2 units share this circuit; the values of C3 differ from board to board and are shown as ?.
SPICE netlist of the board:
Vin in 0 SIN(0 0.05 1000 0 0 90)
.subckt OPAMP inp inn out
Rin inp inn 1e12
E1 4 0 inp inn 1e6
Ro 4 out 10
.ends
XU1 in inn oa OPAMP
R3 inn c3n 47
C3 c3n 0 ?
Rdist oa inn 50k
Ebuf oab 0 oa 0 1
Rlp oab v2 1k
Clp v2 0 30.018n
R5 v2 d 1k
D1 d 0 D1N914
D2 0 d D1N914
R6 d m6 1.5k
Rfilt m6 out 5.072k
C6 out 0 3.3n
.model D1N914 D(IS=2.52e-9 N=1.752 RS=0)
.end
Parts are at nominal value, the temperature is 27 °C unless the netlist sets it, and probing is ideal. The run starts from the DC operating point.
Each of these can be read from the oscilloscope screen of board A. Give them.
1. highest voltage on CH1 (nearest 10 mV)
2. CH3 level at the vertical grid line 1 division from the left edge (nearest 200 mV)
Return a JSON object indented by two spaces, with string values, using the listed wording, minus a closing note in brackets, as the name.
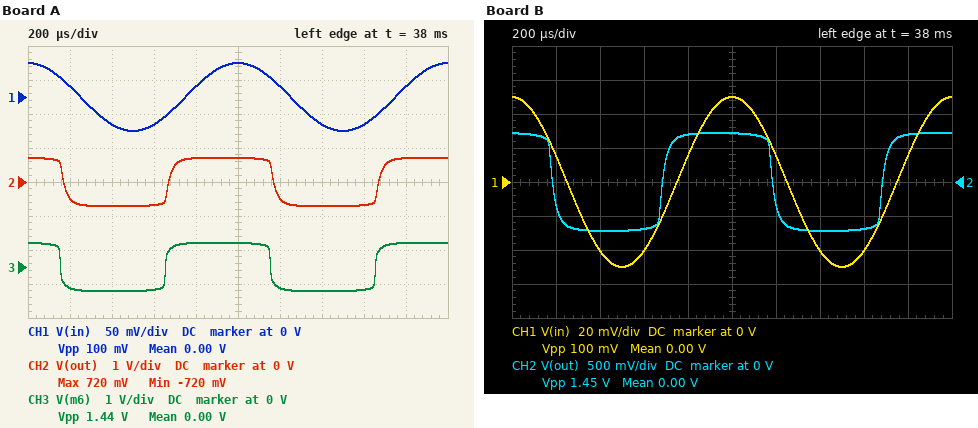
{
  "highest voltage on CH1": "50 mV",
  "CH3 level at the vertical grid line 1 division from the left edge": "-600 mV"
}
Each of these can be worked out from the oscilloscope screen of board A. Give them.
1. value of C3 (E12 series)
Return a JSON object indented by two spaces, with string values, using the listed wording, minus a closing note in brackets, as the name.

{
  "value of C3": "3.9 µF"
}
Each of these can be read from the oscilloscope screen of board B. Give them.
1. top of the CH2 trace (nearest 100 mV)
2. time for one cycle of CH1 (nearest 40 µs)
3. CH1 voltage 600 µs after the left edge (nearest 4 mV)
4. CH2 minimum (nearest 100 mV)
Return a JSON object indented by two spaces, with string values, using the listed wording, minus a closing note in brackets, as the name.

{
  "top of the CH2 trace": "700 mV",
  "time for one cycle of CH1": "1.00 ms",
  "CH1 voltage 600 µs after the left edge": "-40 mV",
  "CH2 minimum": "-700 mV"
}
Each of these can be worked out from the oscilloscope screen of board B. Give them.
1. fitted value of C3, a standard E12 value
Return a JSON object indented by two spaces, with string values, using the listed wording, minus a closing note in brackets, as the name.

{
  "fitted value of C3, a standard E12 value": "4.7 µF"
}
